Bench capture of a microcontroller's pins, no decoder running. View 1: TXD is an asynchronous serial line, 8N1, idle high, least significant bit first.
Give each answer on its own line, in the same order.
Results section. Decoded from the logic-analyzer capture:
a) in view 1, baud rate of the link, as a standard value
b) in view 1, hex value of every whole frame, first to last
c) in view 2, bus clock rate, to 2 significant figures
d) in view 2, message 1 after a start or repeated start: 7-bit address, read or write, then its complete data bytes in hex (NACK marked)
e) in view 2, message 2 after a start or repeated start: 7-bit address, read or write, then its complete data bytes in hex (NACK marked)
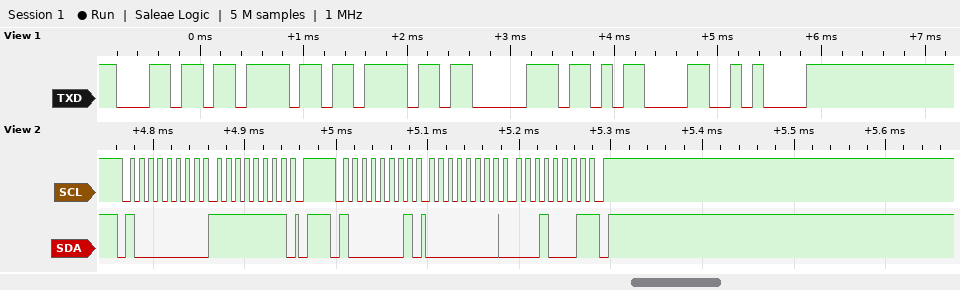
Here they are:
9600 baud
6C 6F 6F 70 0D 0A
100 kHz
0x40 write: FF
0x40 read: 00 11 NACK
